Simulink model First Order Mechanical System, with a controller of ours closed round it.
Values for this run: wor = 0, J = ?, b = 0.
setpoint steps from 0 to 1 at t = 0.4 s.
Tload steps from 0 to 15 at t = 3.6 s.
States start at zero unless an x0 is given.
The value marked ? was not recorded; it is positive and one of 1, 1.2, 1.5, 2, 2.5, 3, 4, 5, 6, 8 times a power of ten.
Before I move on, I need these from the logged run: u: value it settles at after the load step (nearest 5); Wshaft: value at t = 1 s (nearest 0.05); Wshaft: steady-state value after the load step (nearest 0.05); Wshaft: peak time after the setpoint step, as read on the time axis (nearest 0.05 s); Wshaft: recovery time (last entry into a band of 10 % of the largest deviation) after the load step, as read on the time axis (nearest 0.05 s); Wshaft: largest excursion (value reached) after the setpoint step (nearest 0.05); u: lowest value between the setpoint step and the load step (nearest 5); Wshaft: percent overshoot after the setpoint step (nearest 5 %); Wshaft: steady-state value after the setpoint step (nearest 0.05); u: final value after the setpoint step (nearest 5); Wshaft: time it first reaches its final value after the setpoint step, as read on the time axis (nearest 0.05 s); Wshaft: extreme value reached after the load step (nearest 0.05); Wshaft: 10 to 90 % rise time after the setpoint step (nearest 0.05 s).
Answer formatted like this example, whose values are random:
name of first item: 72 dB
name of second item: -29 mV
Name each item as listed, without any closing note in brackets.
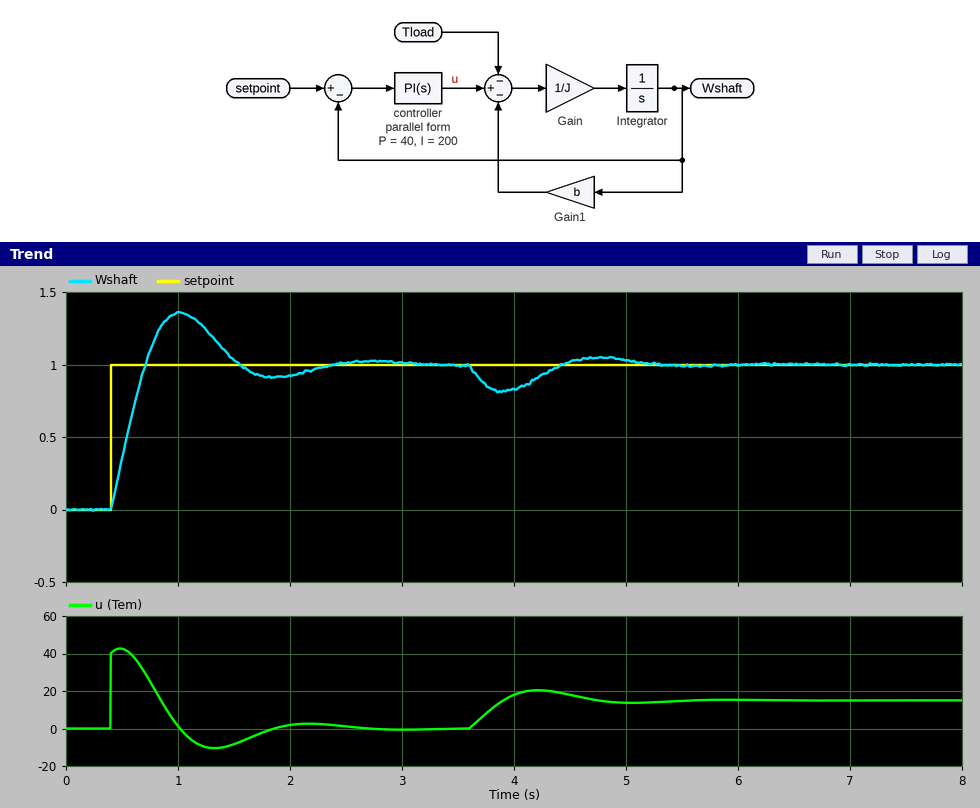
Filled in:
u: value it settles at after the load step: 15
Wshaft: value at t = 1 s: 1.35
Wshaft: steady-state value after the load step: 1.00
Wshaft: peak time after the setpoint step, as read on the time axis: 1.00 s
Wshaft: recovery time (last entry into a band of 10 % of the largest deviation) after the load step, as read on the time axis: 5.10 s
Wshaft: largest excursion (value reached) after the setpoint step: 1.35
u: lowest value between the setpoint step and the load step: -10
Wshaft: percent overshoot after the setpoint step: 35 %
Wshaft: steady-state value after the setpoint step: 1.00
u: final value after the setpoint step: 0
Wshaft: time it first reaches its final value after the setpoint step, as read on the time axis: 0.70 s
Wshaft: extreme value reached after the load step: 0.80
Wshaft: 10 to 90 % rise time after the setpoint step: 0.25 s
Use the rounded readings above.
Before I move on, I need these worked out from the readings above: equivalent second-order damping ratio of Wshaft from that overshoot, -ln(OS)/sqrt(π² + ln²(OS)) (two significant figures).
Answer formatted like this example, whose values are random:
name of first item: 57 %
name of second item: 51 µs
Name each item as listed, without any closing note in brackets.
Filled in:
equivalent second-order damping ratio of Wshaft from that overshoot, -ln(OS)/sqrt(π² + ln²(OS)): 0.32
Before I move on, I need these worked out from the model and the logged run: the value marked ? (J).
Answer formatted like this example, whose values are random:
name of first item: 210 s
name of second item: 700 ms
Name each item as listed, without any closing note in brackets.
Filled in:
the value marked ?: 12
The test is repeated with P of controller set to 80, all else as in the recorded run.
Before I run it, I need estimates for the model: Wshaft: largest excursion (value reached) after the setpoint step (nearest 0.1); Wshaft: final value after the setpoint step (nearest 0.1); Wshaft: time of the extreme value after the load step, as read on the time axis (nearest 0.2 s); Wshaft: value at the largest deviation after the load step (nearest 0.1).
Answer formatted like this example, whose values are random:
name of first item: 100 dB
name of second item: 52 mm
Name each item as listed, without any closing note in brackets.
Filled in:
Wshaft: largest excursion (value reached) after the setpoint step: 1.2
Wshaft: final value after the setpoint step: 1.0
Wshaft: time of the extreme value after the load step, as read on the time axis: 3.8 s
Wshaft: value at the largest deviation after the load step: 0.9
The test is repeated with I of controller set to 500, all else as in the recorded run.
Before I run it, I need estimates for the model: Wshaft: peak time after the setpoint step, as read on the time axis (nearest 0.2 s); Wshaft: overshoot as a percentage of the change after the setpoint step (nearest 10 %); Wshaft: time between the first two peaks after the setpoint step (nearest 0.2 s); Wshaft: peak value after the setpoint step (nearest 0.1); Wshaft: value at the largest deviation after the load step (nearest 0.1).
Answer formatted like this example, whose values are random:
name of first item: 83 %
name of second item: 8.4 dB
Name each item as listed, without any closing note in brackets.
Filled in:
Wshaft: peak time after the setpoint step, as read on the time axis: 0.8 s
Wshaft: overshoot as a percentage of the change after the setpoint step: 50 %
Wshaft: time between the first two peaks after the setpoint step: 1.0 s
Wshaft: peak value after the setpoint step: 1.5
Wshaft: value at the largest deviation after the load step: 0.9
